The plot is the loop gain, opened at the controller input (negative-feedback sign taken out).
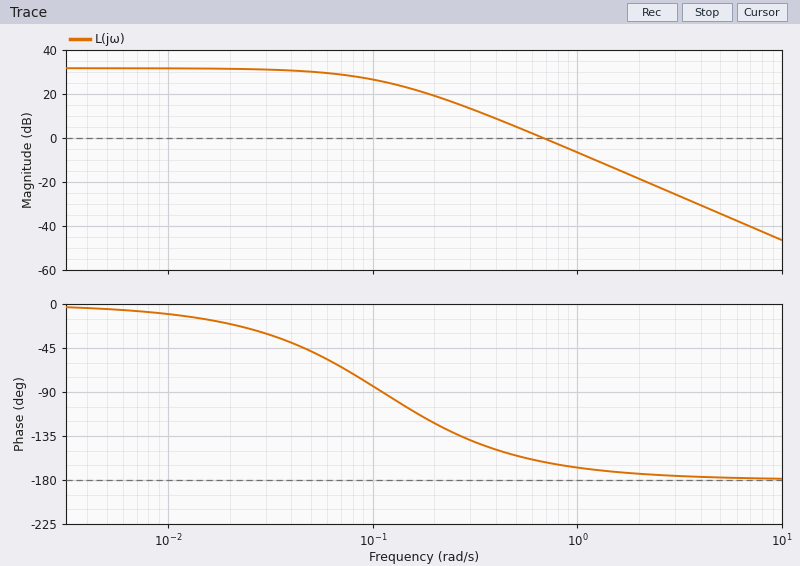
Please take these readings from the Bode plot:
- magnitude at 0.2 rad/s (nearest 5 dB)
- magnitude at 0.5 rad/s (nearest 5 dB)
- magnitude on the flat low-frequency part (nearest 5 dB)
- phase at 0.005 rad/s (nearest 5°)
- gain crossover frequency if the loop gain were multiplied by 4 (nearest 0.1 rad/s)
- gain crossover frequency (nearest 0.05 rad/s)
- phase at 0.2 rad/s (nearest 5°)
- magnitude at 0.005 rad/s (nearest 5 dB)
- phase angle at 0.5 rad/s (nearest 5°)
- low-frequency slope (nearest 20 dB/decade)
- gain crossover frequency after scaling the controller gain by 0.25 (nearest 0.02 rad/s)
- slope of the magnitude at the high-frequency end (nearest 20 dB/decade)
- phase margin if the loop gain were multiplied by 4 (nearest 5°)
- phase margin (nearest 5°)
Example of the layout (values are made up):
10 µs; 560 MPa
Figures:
20 dB; 5 dB; 30 dB; -5°; 1.4 rad/s; 0.70 rad/s; -120°; 30 dB; -155°; 0 dB/decade; 0.32 rad/s; -40 dB/decade; 10°; 20°
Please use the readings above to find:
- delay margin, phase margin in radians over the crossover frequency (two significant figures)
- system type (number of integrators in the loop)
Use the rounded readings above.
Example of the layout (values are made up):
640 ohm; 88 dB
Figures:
0.50 s; 0
